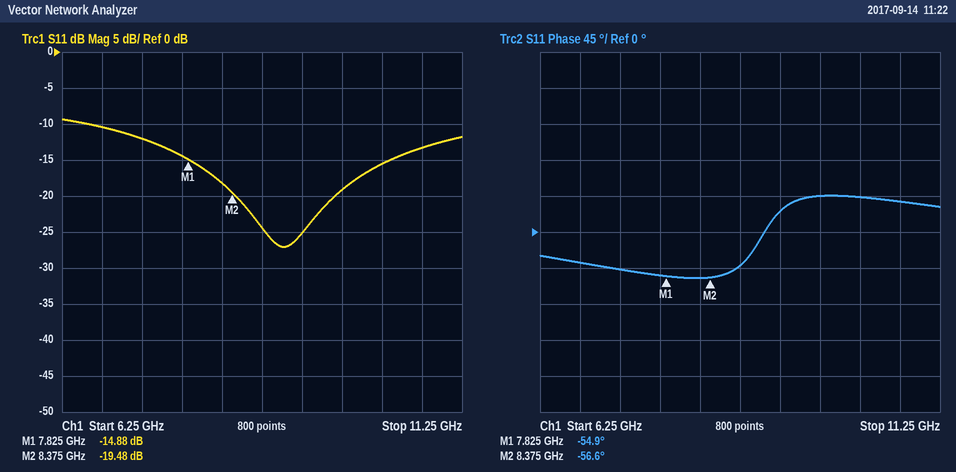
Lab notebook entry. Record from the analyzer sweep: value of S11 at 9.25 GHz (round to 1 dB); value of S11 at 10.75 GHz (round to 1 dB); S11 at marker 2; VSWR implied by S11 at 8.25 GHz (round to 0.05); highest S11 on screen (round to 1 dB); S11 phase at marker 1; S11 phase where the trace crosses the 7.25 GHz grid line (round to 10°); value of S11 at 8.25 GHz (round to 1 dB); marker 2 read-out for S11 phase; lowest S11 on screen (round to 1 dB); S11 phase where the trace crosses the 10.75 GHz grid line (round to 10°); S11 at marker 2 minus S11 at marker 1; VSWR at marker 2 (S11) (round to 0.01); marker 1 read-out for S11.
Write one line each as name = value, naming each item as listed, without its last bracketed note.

value of S11 at 9.25 GHz = -25 dB
value of S11 at 10.75 GHz = -13 dB
S11 at marker 2 = -19.48 dB
VSWR implied by S11 at 8.25 GHz = 1.30
highest S11 on screen = -9 dB
S11 phase at marker 1 = -54.9°
S11 phase where the trace crosses the 7.25 GHz grid line = -50°
value of S11 at 8.25 GHz = -18 dB
marker 2 read-out for S11 phase = -56.6°
lowest S11 on screen = -27 dB
S11 phase where the trace crosses the 10.75 GHz grid line = 40°
S11 at marker 2 minus S11 at marker 1 = -4.60 dB
VSWR at marker 2 (S11) = 1.24
marker 1 read-out for S11 = -14.88 dB
